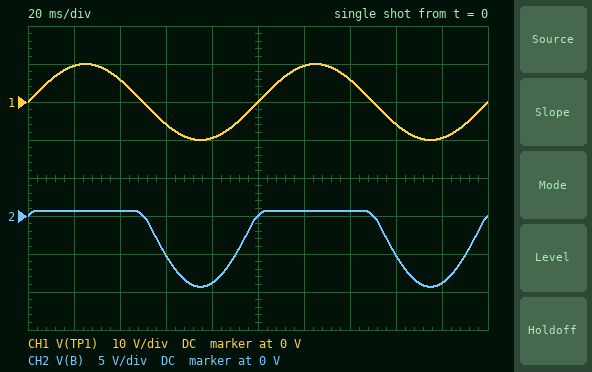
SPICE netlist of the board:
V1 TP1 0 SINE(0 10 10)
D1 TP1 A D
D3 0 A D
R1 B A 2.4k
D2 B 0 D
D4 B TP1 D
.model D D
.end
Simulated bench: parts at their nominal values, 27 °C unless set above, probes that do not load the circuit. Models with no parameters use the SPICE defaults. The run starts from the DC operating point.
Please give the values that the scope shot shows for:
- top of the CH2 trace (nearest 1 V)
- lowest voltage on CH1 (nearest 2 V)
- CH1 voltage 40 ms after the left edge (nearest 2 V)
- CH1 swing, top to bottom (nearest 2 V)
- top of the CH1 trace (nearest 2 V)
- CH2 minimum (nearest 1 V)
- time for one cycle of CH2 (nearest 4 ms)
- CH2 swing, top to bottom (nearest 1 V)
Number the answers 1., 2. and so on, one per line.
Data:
1. 1 V
2. -10 V
3. 6 V
4. 20 V
5. 10 V
6. -9 V
7. 100 ms
8. 10 V
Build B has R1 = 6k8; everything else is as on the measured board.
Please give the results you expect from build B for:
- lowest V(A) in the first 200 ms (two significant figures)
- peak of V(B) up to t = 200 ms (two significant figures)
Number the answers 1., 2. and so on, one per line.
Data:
1. -660 mV
2. 660 mV
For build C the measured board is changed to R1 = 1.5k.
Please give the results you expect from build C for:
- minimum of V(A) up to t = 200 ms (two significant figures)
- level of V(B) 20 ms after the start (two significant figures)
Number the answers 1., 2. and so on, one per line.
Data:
1. -700 mV
2. 700 mV
